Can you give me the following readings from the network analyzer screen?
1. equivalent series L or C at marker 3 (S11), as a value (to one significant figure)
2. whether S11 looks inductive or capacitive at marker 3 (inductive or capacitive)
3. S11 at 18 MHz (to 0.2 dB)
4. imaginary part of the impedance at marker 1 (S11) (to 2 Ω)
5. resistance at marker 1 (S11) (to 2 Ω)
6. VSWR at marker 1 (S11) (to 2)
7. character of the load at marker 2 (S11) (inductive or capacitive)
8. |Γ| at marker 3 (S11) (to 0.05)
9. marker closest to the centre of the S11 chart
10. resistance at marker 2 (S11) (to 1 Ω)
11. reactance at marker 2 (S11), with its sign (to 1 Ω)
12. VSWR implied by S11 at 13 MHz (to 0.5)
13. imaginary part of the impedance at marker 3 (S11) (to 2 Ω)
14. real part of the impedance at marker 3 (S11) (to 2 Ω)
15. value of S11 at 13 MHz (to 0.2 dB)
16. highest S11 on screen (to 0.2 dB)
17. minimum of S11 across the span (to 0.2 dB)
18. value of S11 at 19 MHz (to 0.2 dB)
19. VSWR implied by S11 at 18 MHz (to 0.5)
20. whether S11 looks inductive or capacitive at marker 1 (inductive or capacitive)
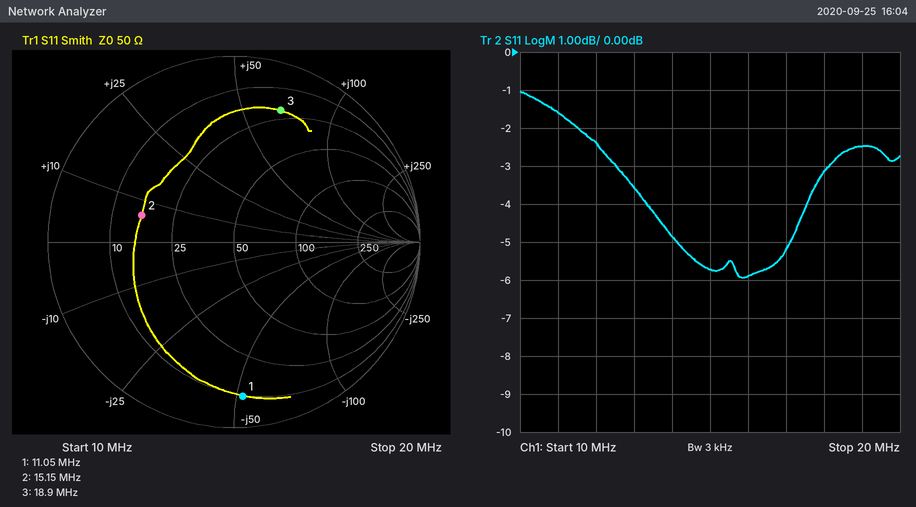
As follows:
600 nH
inductive
-3.2 dB
-52 Ω
10 Ω
10
inductive
0.75
marker 2
16 Ω
+6 Ω
5.0
+66 Ω
20 Ω
-3.6 dB
-1.0 dB
-6.0 dB
-2.4 dB
5.5
capacitive
